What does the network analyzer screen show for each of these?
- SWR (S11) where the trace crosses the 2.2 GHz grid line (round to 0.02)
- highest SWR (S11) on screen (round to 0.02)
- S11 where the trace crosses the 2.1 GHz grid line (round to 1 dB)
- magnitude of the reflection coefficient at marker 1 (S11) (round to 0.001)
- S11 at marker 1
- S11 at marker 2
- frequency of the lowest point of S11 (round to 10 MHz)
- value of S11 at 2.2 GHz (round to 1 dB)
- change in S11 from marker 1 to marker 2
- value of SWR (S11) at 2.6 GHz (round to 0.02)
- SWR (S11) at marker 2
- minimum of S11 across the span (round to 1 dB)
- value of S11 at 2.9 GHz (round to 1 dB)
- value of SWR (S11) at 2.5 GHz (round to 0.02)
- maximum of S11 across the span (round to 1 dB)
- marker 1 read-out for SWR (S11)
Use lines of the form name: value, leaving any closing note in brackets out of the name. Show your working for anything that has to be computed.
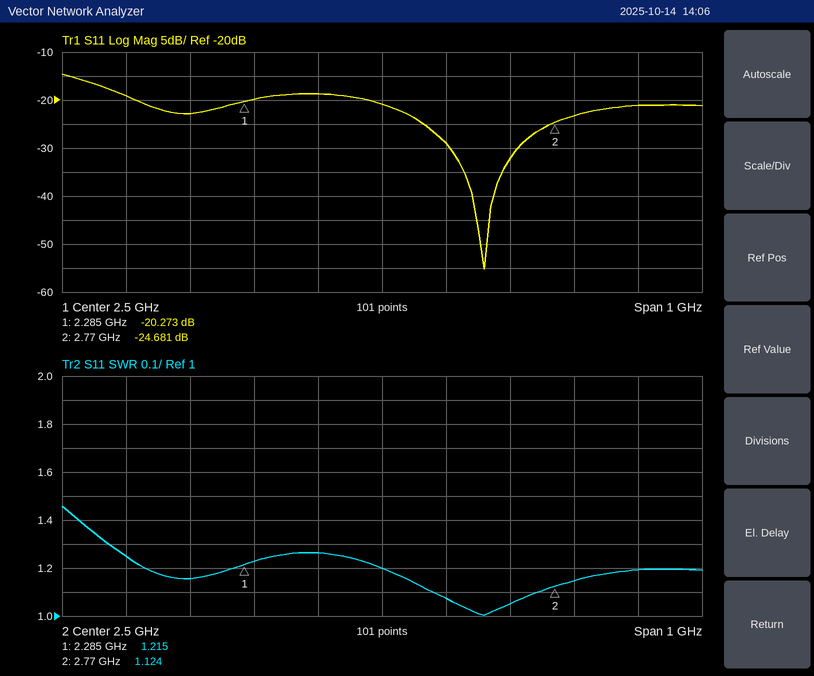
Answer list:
SWR (S11) where the trace crosses the 2.2 GHz grid line: 1.16
highest SWR (S11) on screen: 1.46
S11 where the trace crosses the 2.1 GHz grid line: -19 dB
magnitude of the reflection coefficient at marker 1 (S11): 10^(-20.273/20) ≈ 0.097
S11 at marker 1: -20.273 dB
S11 at marker 2: -24.681 dB
frequency of the lowest point of S11: 2.66 GHz
value of S11 at 2.2 GHz: -23 dB
change in S11 from marker 1 to marker 2: -24.681 − (-20.273) = -4.408 dB
value of SWR (S11) at 2.6 GHz: 1.08
SWR (S11) at marker 2: 1.124
minimum of S11 across the span: -55 dB
value of S11 at 2.9 GHz: -21 dB
value of SWR (S11) at 2.5 GHz: 1.20
maximum of S11 across the span: -15 dB
marker 1 read-out for SWR: 1.215
